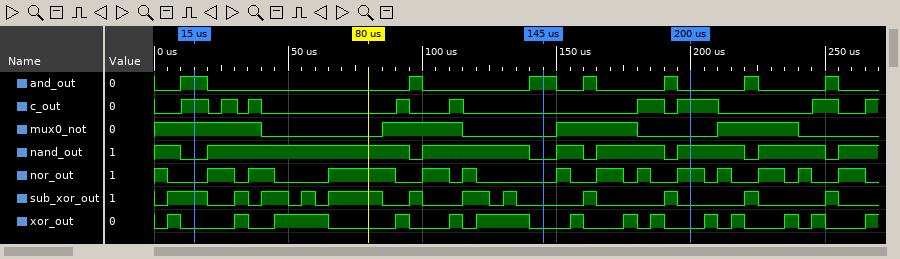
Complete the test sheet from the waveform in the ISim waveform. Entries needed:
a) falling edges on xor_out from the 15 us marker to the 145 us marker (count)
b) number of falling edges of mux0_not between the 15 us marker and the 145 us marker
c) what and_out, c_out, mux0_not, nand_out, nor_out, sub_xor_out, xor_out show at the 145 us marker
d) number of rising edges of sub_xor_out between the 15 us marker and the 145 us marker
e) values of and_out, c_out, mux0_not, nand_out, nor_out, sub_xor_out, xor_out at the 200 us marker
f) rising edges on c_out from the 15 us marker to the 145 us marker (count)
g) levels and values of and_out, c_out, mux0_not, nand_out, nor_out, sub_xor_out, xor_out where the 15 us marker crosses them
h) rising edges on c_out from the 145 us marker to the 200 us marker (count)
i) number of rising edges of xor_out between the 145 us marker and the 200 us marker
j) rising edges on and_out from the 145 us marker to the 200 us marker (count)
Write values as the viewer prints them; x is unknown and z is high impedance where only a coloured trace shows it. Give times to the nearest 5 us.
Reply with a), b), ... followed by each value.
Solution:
a) 5
b) 2
c) and_out=1, c_out=0, mux0_not=0, nand_out=0, nor_out=0, sub_xor_out=0, xor_out=0
d) 7
e) and_out=0, c_out=1, mux0_not=0, nand_out=1, nor_out=1, sub_xor_out=0, xor_out=0
f) 4
g) and_out=1, c_out=1, mux0_not=1, nand_out=0, nor_out=0, sub_xor_out=1, xor_out=0
h) 2
i) 3
j) 2
